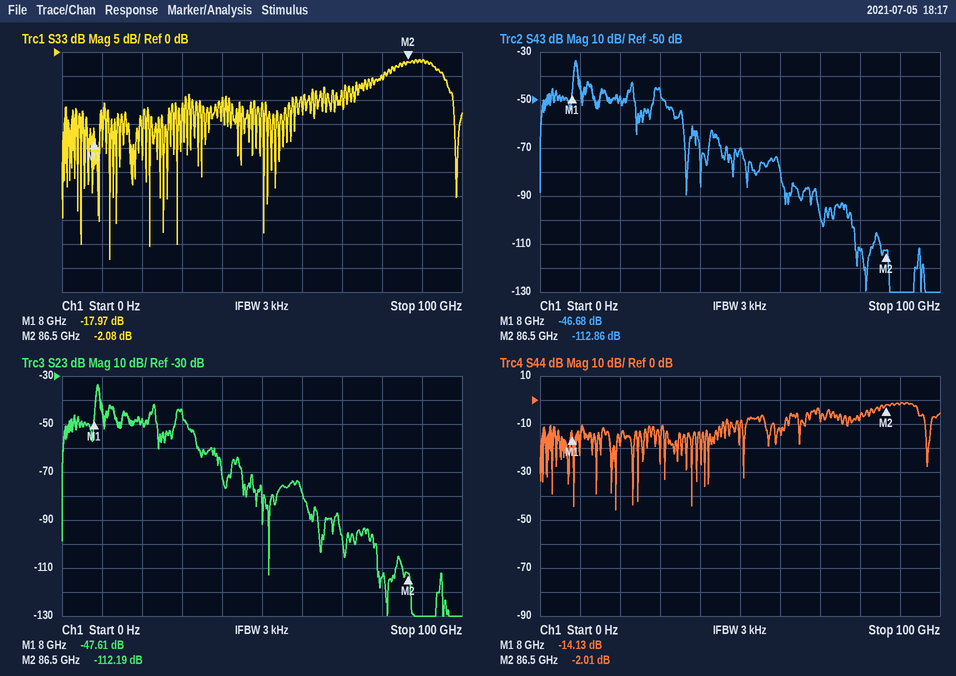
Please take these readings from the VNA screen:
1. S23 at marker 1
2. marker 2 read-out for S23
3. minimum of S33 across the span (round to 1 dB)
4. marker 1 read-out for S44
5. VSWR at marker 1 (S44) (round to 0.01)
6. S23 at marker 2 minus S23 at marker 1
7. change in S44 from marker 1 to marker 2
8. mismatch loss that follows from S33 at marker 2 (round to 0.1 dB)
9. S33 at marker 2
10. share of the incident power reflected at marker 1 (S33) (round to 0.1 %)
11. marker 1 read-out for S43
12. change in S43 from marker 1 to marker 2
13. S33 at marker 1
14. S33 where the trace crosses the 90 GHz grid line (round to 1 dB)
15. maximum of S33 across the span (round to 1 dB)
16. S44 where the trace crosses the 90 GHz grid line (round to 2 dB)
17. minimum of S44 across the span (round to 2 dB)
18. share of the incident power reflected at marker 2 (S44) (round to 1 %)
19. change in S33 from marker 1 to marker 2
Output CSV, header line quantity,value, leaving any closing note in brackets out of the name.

quantity,value
S23 at marker 1,-47.61 dB
marker 2 read-out for S23,-112.19 dB
minimum of S33 across the span,-43 dB
marker 1 read-out for S44,-14.13 dB
VSWR at marker 1 (S44),1.49
S23 at marker 2 minus S23 at marker 1,-64.58 dB
change in S44 from marker 1 to marker 2,12.12 dB
mismatch loss that follows from S33 at marker 2,4.2 dB
S33 at marker 2,-2.08 dB
share of the incident power reflected at marker 1 (S33),1.6 %
marker 1 read-out for S43,-46.68 dB
change in S43 from marker 1 to marker 2,-66.18 dB
S33 at marker 1,-17.97 dB
S33 where the trace crosses the 90 GHz grid line,-2 dB
maximum of S33 across the span,-2 dB
S44 where the trace crosses the 90 GHz grid line,-2 dB
minimum of S44 across the span,-46 dB
share of the incident power reflected at marker 2 (S44),63 %
change in S33 from marker 1 to marker 2,15.89 dB
